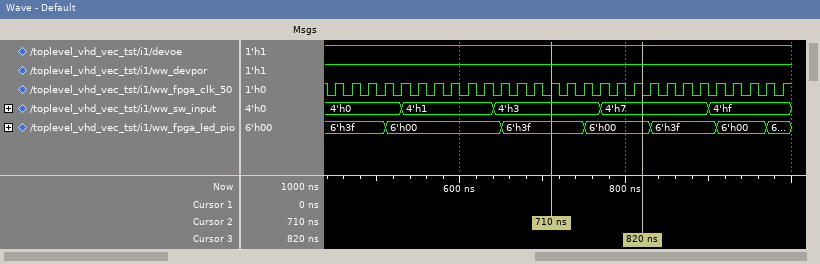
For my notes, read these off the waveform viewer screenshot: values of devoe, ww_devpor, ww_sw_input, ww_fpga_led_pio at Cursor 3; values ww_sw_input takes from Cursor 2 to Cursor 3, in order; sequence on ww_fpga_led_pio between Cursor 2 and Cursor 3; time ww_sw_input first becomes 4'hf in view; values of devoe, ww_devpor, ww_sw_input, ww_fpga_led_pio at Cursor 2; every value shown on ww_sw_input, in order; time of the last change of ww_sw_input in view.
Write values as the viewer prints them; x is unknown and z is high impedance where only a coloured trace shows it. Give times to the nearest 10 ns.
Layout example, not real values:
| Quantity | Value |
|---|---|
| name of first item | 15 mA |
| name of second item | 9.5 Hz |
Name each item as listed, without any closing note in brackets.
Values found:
| Quantity | Value |
|---|---|
| values of devoe, ww_devpor, ww_sw_input, ww_fpga_led_pio at Cursor 3 | devoe=1, ww_devpor=1, ww_sw_input=4'h7, ww_fpga_led_pio=6'h00 |
| values ww_sw_input takes from Cursor 2 to Cursor 3, in order | 4'h3, 4'h7 |
| sequence on ww_fpga_led_pio between Cursor 2 and Cursor 3 | 6'h3f, 6'h00 |
| time ww_sw_input first becomes 4'hf in view | 900 ns |
| values of devoe, ww_devpor, ww_sw_input, ww_fpga_led_pio at Cursor 2 | devoe=1, ww_devpor=1, ww_sw_input=4'h3, ww_fpga_led_pio=6'h3f |
| every value shown on ww_sw_input, in order | 4'h0, 4'h1, 4'h3, 4'h7, 4'hf |
| time of the last change of ww_sw_input in view | 900 ns |
